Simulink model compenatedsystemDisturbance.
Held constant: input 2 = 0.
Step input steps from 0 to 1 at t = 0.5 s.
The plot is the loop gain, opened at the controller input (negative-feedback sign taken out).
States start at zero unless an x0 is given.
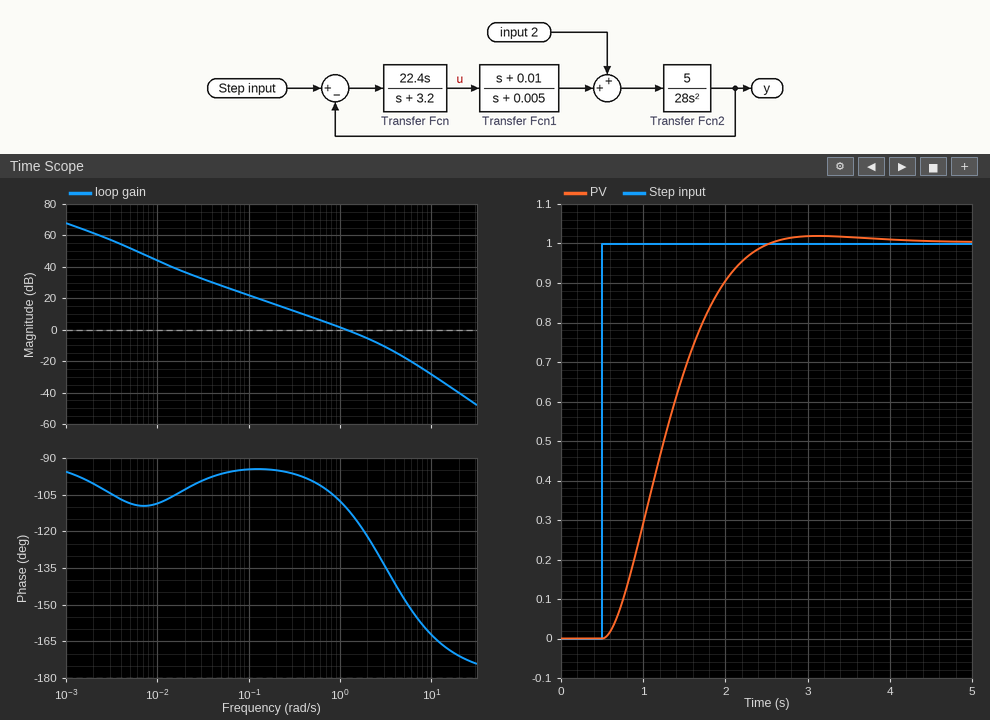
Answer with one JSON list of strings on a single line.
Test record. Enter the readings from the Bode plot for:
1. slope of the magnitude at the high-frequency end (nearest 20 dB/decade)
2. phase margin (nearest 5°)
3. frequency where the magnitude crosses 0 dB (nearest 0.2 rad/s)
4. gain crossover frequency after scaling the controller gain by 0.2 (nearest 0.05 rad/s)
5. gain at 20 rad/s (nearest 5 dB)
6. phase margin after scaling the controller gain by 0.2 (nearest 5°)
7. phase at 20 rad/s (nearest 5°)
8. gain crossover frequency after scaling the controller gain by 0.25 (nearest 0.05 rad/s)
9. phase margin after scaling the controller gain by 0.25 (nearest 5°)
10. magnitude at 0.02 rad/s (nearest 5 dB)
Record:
["-40 dB/decade", "70°", "1.2 rad/s", "0.25 rad/s", "-40 dB", "85°", "-170°", "0.30 rad/s", "85°", "35 dB"]
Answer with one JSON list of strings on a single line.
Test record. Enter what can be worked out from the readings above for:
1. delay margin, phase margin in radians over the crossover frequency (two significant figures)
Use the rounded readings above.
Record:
["1.0 s"]
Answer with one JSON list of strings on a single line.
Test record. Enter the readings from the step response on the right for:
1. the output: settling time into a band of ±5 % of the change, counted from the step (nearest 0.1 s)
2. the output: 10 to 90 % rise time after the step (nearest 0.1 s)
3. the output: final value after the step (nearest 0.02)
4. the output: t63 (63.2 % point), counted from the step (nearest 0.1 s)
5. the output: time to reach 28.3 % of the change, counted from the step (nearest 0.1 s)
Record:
["1.7 s", "1.2 s", "1.00", "0.9 s", "0.5 s"]
